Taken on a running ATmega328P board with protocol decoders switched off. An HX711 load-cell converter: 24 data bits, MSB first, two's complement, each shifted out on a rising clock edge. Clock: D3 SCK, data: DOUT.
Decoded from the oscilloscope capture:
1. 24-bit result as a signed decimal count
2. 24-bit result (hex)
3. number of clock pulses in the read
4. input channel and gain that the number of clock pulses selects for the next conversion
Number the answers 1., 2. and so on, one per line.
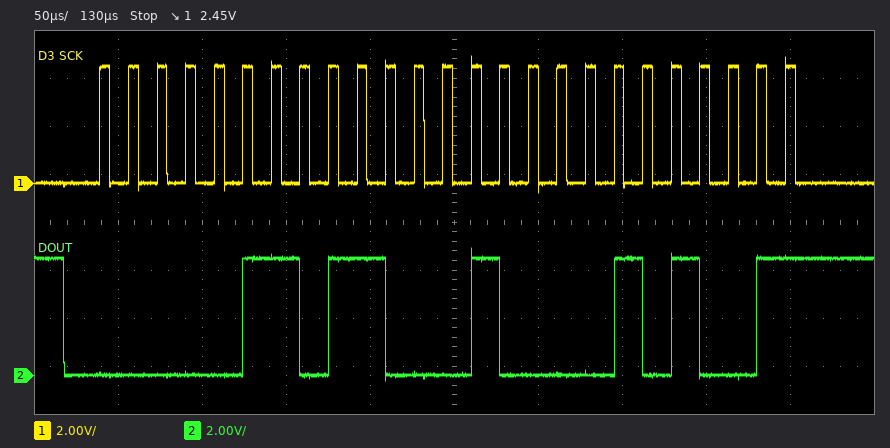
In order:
1. 443433
2. 0x06C429
3. 25
4. channel A, gain 128
